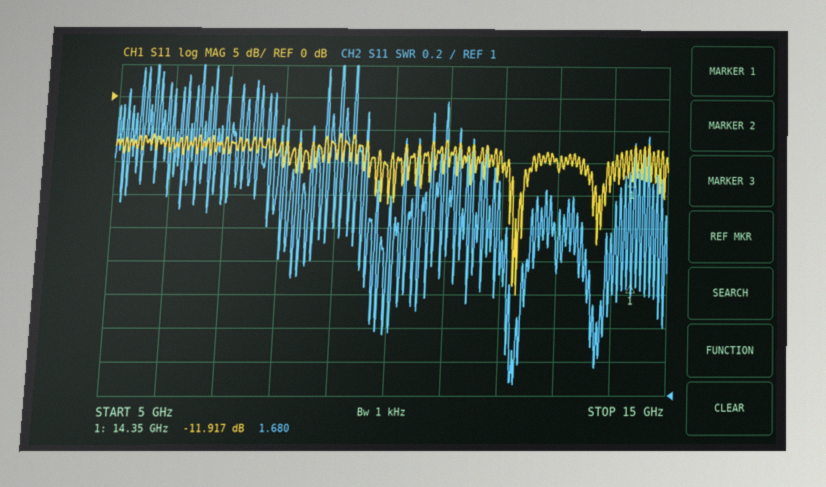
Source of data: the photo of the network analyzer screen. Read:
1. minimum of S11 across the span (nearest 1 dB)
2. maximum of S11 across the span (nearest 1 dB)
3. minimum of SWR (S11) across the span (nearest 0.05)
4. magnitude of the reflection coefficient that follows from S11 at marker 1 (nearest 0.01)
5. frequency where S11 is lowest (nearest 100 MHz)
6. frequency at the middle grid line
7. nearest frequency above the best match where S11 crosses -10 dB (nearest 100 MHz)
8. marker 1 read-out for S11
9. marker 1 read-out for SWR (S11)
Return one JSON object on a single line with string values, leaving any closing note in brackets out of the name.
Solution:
{"minimum of S11 across the span": "-30 dB", "maximum of S11 across the span": "-6 dB", "minimum of SWR (S11) across the span": "1.05", "magnitude of the reflection coefficient that follows from S11 at marker 1": "0.25", "frequency where S11 is lowest": "12.3 GHz", "frequency at the middle grid line": "10 GHz", "nearest frequency above the best match where S11 crosses -10 dB": "12.5 GHz", "marker 1 read-out for S11": "-11.917 dB", "marker 1 read-out for SWR": "1.680"}
